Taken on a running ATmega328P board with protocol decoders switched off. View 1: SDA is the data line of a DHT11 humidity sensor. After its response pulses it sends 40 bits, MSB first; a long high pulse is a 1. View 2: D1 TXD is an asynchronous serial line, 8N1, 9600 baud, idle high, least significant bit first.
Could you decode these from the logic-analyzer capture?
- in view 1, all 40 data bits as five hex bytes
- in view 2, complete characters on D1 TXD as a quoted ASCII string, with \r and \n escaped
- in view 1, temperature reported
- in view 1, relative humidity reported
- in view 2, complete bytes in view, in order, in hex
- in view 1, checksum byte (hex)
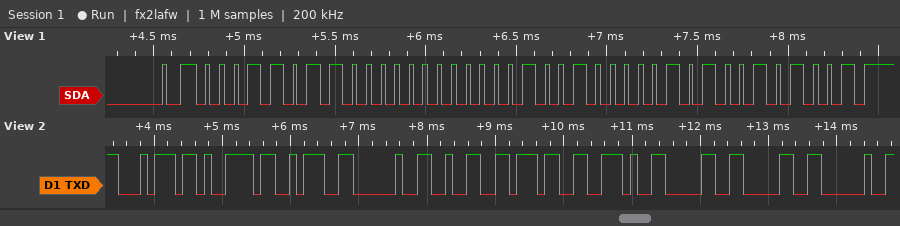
1B 00 09 05 29
"ty: 27.00 "
9.5 °C
27 %
74 79 3A 20 32 37 2E 30 30 20
0x29
